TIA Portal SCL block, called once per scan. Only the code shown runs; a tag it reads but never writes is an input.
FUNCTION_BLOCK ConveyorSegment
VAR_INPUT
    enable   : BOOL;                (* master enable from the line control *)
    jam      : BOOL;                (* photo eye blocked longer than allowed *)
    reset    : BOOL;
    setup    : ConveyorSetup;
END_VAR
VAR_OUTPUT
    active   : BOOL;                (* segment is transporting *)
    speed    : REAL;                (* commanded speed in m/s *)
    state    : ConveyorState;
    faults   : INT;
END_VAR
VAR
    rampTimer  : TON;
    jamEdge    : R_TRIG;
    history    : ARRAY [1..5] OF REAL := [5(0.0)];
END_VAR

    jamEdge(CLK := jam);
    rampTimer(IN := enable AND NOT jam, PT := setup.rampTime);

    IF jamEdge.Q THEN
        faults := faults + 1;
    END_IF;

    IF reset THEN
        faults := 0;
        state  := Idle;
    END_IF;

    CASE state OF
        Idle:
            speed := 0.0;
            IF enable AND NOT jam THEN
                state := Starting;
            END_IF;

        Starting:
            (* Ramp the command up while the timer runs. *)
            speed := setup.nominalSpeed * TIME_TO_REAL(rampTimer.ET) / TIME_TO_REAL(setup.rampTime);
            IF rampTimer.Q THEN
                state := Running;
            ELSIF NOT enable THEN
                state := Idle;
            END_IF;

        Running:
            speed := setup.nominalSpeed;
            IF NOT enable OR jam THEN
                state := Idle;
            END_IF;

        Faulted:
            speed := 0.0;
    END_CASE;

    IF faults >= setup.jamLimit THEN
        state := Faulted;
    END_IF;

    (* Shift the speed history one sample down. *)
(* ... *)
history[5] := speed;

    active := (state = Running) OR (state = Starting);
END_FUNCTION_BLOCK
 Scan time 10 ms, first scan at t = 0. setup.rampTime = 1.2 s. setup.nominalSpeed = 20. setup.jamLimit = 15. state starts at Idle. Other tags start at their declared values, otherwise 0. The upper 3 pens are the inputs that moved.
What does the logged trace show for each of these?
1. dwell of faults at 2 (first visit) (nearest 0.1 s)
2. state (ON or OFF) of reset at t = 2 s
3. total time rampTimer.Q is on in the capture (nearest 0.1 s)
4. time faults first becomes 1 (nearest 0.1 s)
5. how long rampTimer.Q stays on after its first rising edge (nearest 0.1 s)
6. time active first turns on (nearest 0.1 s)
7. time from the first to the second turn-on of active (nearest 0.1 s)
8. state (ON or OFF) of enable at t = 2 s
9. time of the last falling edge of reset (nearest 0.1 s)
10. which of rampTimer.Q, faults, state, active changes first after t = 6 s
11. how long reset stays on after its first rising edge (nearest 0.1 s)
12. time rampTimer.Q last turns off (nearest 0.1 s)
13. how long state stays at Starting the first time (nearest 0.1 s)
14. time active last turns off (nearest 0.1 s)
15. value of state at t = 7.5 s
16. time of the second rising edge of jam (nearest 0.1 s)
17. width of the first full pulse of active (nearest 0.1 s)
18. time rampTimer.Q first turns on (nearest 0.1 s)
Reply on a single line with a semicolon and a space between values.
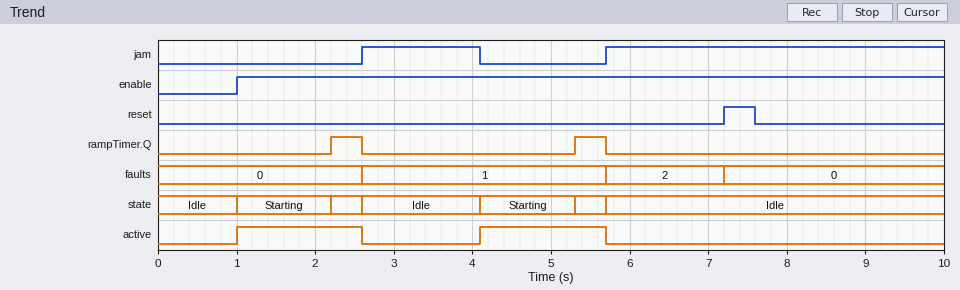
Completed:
1.5 s; OFF; 0.8 s; 2.6 s; 0.4 s; 1.0 s; 3.1 s; ON; 7.6 s; faults; 0.4 s; 5.7 s; 1.2 s; 5.7 s; Idle; 5.7 s; 1.6 s; 2.2 s
